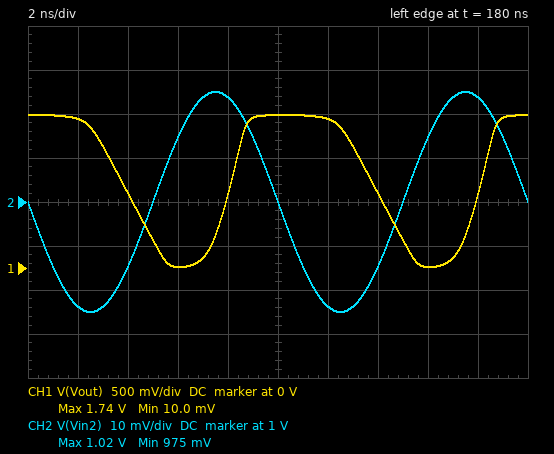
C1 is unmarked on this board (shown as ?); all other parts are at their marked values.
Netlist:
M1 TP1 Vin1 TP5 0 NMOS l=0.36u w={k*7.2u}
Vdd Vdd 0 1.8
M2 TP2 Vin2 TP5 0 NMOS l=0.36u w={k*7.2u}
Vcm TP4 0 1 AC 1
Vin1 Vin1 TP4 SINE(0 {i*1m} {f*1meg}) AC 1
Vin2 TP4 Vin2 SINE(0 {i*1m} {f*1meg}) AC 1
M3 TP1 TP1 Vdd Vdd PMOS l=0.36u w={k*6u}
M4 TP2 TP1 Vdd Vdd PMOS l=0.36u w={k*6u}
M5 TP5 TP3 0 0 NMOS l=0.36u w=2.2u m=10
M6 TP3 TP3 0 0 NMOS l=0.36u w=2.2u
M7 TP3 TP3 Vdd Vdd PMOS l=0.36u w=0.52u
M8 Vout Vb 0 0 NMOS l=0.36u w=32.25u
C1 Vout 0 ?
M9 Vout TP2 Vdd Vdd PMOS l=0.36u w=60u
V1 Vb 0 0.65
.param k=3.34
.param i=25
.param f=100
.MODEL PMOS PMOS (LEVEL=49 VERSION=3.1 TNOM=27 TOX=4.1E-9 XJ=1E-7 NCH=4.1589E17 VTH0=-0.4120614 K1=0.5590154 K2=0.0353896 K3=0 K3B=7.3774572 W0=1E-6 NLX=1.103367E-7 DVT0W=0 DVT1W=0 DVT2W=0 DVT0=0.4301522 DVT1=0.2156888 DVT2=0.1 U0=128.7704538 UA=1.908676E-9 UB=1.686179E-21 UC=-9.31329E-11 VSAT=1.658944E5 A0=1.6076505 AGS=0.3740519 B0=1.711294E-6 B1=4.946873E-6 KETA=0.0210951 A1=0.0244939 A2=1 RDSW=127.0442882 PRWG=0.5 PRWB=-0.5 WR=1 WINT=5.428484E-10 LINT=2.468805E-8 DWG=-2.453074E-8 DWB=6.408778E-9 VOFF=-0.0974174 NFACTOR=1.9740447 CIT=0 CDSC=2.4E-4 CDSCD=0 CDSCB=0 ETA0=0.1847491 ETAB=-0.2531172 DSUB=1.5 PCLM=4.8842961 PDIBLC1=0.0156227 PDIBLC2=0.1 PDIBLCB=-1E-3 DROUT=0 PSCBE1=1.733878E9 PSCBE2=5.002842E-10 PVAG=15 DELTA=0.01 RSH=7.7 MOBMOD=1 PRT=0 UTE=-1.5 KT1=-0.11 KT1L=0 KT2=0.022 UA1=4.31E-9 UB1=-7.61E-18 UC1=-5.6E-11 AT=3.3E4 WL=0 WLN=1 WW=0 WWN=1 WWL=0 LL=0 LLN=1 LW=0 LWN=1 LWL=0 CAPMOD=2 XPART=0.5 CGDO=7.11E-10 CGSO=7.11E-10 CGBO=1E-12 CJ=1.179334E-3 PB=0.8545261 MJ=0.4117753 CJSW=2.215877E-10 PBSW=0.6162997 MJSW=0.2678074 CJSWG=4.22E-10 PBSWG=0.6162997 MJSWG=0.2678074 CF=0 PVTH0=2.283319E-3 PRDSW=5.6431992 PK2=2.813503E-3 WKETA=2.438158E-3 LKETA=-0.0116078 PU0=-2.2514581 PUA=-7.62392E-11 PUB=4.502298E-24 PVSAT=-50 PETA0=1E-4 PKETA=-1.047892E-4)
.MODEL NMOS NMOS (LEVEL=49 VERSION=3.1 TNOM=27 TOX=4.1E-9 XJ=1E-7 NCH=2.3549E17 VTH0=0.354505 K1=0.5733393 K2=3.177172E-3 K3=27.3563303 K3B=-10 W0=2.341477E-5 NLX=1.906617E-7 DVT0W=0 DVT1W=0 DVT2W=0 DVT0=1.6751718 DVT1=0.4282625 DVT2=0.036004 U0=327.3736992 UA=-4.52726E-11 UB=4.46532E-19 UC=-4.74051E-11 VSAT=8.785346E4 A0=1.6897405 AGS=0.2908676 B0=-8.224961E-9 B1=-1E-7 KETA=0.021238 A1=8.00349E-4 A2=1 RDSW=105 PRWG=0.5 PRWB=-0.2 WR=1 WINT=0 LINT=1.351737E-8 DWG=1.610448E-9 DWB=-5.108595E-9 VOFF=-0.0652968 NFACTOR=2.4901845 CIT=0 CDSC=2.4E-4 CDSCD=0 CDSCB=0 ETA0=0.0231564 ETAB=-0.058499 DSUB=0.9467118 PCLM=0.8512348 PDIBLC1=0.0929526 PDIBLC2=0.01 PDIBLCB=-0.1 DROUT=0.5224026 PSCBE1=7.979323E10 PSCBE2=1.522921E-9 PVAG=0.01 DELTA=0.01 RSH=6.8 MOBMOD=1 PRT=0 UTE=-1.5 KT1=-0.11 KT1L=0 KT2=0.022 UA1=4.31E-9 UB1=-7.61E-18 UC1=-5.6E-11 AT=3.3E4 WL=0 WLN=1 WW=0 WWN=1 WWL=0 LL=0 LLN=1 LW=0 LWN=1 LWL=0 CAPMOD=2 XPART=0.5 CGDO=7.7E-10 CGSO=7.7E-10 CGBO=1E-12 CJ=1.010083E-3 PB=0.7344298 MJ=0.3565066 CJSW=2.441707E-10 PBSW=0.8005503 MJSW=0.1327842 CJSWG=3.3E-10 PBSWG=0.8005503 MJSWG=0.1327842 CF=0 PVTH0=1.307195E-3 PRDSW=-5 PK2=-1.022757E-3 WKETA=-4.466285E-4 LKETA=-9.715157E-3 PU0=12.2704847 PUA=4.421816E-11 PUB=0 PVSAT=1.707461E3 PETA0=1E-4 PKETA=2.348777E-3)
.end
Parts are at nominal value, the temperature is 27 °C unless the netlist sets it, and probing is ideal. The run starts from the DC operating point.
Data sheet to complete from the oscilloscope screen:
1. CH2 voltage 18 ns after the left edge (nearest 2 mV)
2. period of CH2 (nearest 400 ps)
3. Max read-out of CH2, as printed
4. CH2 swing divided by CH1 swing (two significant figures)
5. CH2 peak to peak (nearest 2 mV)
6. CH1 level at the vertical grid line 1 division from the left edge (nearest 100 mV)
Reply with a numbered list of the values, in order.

1. 1.024 V
2. 10.0 ns
3. 1.02 V
4. 0.029
5. 50 mV
6. 1.7 V
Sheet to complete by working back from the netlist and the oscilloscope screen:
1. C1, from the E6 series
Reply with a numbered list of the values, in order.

1. 470 fF
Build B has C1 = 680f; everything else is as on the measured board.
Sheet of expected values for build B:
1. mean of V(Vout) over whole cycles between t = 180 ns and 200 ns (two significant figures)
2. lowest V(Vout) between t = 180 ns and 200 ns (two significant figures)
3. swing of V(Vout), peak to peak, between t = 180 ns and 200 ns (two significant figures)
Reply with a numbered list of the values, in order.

1. 1.1 V
2. 140 mV
3. 1.6 V
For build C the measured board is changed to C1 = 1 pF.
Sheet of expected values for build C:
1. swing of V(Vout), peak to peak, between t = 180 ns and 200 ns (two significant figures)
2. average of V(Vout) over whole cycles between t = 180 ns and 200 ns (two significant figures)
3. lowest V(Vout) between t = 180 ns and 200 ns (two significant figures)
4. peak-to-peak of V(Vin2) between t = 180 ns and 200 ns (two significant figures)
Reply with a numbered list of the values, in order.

1. 1.2 V
2. 1.3 V
3. 530 mV
4. 50 mV
